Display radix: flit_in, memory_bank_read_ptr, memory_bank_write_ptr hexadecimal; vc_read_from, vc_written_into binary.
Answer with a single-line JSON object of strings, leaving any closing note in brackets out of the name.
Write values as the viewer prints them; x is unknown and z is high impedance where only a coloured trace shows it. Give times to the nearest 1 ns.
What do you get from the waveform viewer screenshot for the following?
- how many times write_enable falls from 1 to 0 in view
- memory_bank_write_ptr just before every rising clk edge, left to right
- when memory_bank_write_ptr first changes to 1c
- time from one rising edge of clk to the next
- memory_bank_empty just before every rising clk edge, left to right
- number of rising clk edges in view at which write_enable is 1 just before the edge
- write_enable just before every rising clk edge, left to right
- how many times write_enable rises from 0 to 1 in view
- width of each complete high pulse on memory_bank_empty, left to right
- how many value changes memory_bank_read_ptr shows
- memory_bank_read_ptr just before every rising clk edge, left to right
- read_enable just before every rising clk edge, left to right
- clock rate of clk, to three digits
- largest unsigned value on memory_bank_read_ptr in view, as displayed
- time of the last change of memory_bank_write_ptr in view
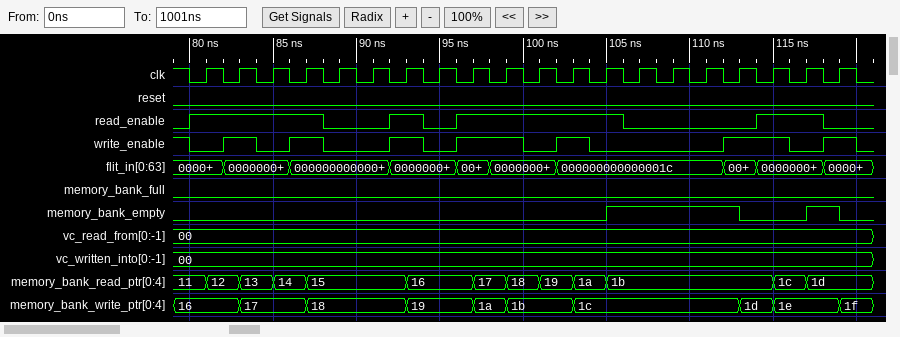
{"how many times write_enable falls from 1 to 0 in view": "8", "memory_bank_write_ptr just before every rising clk edge, left to right": "16, 16, 17, 17, 18, 18, 18, 19, 19, 1a, 1b, 1b, 1c, 1c, 1c, 1c, 1c, 1d, 1e, 1e", "when memory_bank_write_ptr first changes to 1c": "103 ns", "time from one rising edge of clk to the next": "2 ns", "memory_bank_empty just before every rising clk edge, left to right": "0 0 0 0 0 0 0 0 0 0 0 0 0 1 1 1 1 0 0 1", "number of rising clk edges in view at which write_enable is 1 just before the edge": "9", "write_enable just before every rising clk edge, left to right": "0 1 0 1 0 0 1 0 1 1 0 1 0 0 0 0 1 1 0 1", "how many times write_enable rises from 0 to 1 in view": "7", "width of each complete high pulse on memory_bank_empty, left to right": "8 ns, 2 ns", "how many value changes memory_bank_read_ptr shows": "12", "memory_bank_read_ptr just before every rising clk edge, left to right": "11, 12, 13, 14, 15, 15, 15, 16, 16, 17, 18, 19, 1a, 1b, 1b, 1b, 1b, 1b, 1c, 1d", "read_enable just before every rising clk edge, left to right": "1 1 1 1 0 0 1 0 1 1 1 1 1 0 0 0 0 1 1 0", "clock rate of clk, to three digits": "500 MHz", "largest unsigned value on memory_bank_read_ptr in view, as displayed": "1d", "time of the last change of memory_bank_write_ptr in view": "119 ns"}
